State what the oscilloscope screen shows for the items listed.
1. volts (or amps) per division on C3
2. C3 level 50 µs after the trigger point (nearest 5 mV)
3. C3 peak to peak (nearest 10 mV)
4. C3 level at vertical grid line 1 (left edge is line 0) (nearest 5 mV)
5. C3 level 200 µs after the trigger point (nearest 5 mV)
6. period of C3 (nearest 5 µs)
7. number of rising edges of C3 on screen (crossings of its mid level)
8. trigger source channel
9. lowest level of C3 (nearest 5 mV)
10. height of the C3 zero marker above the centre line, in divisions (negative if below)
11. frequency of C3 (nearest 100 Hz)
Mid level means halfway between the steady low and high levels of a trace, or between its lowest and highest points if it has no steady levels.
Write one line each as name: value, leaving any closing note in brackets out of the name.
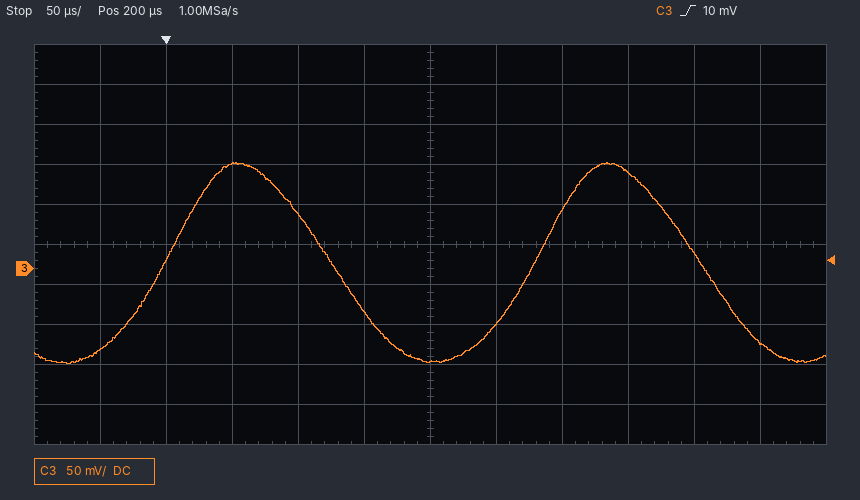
volts (or amps) per division on C3: 50 mV
C3 level 50 µs after the trigger point: 130 mV
C3 peak to peak: 250 mV
C3 level at vertical grid line 1 (left edge is line 0): -100 mV
C3 level 200 µs after the trigger point: -115 mV
period of C3: 280 µs
number of rising edges of C3 on screen: 2
trigger source channel: C3
lowest level of C3: -120 mV
height of the C3 zero marker above the centre line, in divisions: -0.6 div
frequency of C3: 3.6 kHz
